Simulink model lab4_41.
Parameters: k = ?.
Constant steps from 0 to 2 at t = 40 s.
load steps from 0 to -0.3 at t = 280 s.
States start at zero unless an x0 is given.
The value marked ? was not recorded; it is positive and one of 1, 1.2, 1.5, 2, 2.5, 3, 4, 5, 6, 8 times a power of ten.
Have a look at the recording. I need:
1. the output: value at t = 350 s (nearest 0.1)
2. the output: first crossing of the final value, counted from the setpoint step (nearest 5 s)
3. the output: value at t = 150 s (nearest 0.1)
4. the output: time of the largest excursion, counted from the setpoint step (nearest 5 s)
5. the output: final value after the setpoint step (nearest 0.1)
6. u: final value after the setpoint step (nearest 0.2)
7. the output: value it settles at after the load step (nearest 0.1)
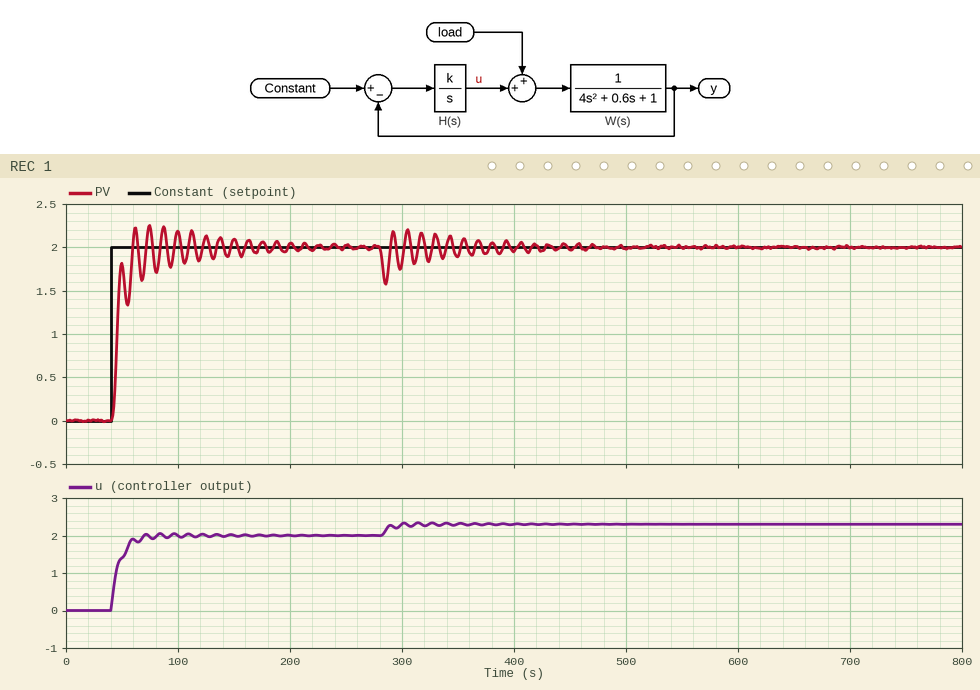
1.9
20 s
2.1
35 s
2.0
2.0
2.0
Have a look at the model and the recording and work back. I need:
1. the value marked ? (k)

0.12
